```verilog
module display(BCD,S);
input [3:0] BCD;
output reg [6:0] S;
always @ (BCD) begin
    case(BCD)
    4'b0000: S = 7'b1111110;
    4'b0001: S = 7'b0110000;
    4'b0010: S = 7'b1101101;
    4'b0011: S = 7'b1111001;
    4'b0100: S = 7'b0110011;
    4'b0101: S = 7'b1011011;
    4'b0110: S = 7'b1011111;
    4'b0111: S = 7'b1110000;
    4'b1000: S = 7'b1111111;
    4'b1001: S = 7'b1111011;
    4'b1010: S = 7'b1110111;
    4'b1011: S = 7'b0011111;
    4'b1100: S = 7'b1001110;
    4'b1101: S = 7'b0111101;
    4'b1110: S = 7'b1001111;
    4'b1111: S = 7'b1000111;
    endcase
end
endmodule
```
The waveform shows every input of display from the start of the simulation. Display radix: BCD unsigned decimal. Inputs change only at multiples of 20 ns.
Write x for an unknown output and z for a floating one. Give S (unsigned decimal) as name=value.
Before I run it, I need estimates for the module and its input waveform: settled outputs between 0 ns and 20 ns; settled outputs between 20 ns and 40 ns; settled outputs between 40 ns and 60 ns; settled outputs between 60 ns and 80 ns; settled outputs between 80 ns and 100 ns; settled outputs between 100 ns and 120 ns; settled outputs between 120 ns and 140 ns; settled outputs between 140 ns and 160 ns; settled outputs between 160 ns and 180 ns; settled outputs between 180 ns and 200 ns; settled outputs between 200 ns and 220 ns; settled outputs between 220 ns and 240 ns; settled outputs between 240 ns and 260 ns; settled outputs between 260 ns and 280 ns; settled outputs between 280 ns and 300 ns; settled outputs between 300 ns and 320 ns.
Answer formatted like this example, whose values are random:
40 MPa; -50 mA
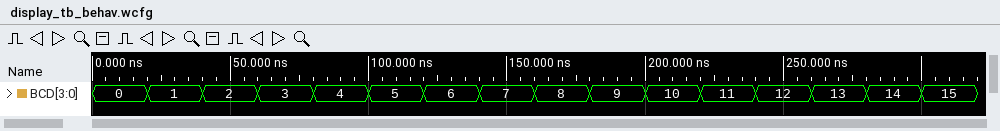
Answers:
S=126; S=48; S=109; S=121; S=51; S=91; S=95; S=112; S=127; S=123; S=119; S=31; S=78; S=61; S=79; S=71
